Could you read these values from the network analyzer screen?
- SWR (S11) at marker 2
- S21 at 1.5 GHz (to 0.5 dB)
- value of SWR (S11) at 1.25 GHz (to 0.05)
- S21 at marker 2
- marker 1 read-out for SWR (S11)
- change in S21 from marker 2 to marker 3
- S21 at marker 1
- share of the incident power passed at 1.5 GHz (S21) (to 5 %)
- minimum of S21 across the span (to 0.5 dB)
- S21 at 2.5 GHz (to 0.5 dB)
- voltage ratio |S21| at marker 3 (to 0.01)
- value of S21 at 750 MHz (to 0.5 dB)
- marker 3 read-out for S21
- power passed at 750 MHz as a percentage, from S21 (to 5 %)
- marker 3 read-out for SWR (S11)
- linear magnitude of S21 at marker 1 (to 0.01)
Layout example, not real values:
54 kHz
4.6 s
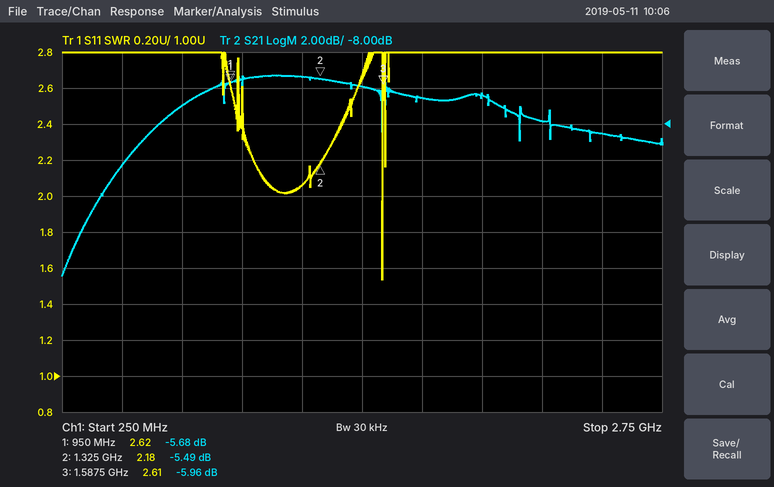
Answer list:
2.18
-6.0 dB
2.05
-5.49 dB
2.62
-0.47 dB
-5.68 dB
25 %
-16.5 dB
-8.5 dB
0.50
-7.0 dB
-5.96 dB
20 %
2.61
0.52
